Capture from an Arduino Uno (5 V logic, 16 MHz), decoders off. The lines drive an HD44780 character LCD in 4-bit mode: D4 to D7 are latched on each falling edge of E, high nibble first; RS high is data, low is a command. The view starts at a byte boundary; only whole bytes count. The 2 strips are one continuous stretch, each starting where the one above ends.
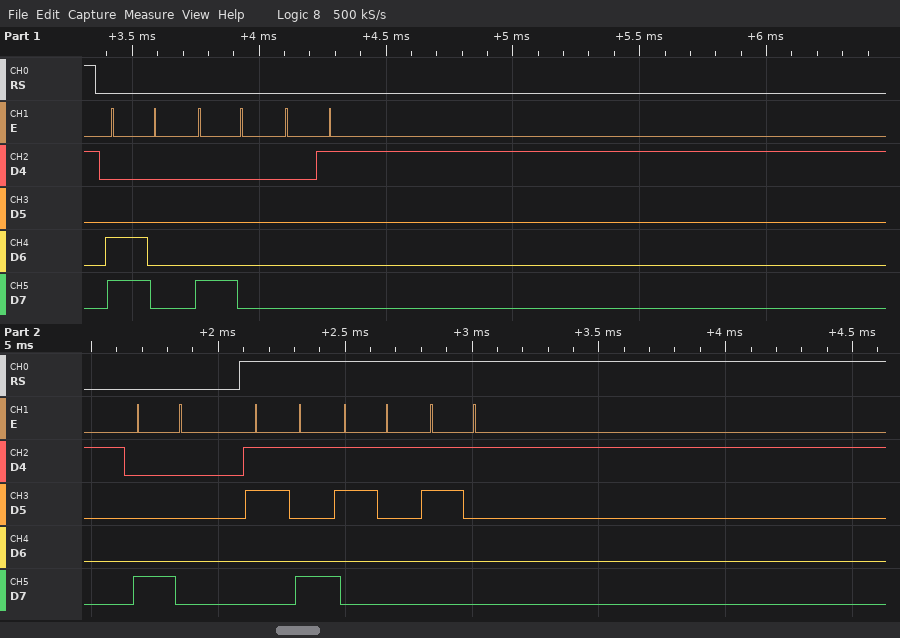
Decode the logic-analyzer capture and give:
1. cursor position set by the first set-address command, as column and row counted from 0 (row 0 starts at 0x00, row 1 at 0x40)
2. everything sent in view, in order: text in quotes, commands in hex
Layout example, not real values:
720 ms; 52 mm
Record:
column 0, row 1; 0xC0 0x80 0x01 0x80 "911"
